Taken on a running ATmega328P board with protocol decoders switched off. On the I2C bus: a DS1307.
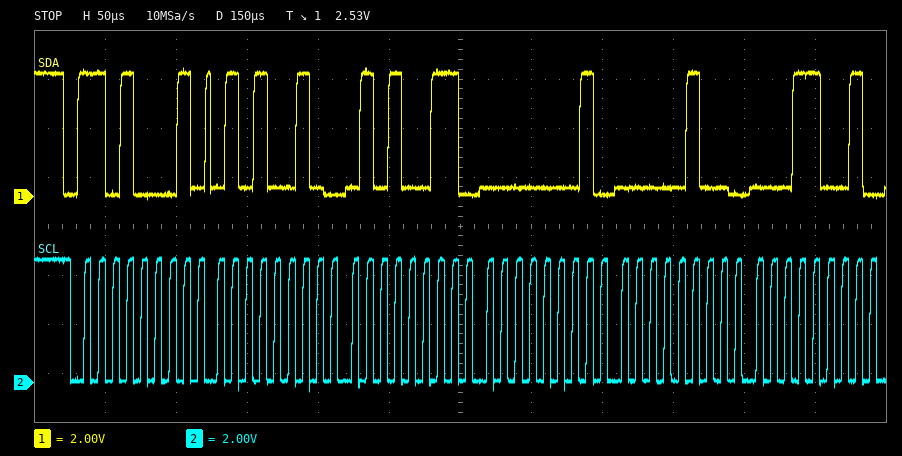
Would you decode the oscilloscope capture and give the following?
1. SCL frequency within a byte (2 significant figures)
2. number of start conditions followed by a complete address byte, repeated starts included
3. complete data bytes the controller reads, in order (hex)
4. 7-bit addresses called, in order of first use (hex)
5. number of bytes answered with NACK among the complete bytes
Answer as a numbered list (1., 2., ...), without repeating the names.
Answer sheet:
1. 100 kHz
2. 1
3. 52 53 01 04 19
4. 0x68
5. 0
